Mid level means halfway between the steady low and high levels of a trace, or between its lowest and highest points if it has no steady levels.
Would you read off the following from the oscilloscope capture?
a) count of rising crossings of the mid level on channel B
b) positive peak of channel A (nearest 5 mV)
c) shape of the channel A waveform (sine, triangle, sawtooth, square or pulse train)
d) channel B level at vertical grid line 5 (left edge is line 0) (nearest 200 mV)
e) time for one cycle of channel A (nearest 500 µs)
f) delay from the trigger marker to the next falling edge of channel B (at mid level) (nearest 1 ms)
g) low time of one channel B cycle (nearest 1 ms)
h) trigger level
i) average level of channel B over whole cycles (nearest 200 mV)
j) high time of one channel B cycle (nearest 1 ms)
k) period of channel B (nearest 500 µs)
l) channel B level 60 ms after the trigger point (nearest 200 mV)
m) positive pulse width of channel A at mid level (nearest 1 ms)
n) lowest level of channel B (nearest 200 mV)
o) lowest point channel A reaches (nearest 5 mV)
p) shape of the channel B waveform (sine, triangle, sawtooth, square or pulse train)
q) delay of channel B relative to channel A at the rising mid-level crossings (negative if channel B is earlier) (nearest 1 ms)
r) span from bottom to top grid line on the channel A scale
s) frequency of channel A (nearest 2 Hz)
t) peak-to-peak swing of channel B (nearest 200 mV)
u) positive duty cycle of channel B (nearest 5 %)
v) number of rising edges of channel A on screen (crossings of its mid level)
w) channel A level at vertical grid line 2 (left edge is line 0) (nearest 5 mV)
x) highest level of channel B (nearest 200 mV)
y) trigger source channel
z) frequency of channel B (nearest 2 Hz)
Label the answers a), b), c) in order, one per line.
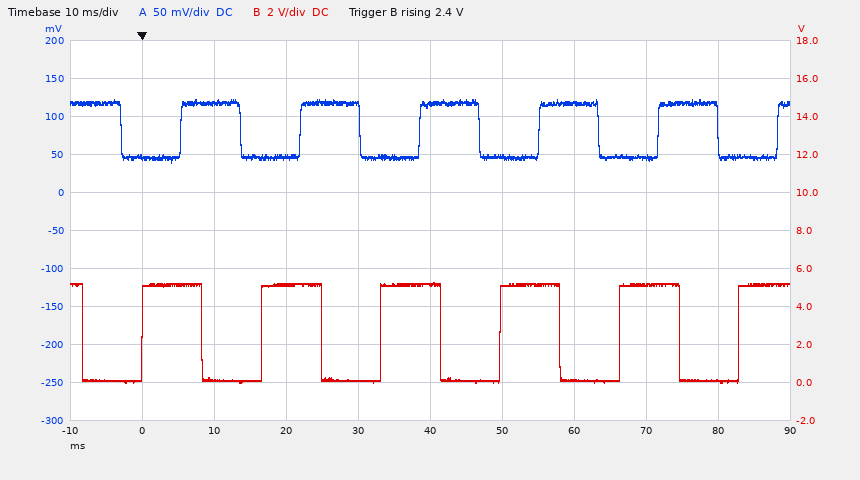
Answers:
a) 6
b) 120 mV
c) square
d) 5.2 V
e) 16.5 ms
f) 8 ms
g) 8 ms
h) 2.4 V
i) 2.6 V
j) 8 ms
k) 16.5 ms
l) 200 mV
m) 8 ms
n) 0.0 V
o) 40 mV
p) square
q) -5 ms
r) 500 mV
s) 60 Hz
t) 5.2 V
u) 50 %
v) 6
w) 115 mV
x) 5.2 V
y) channel B
z) 60 Hz
